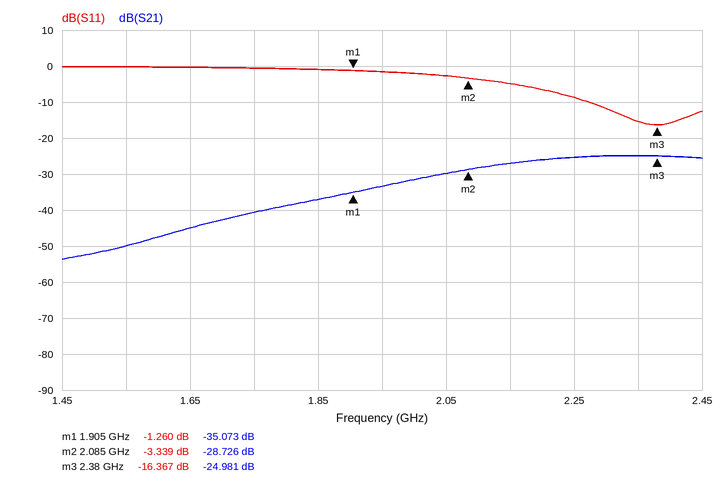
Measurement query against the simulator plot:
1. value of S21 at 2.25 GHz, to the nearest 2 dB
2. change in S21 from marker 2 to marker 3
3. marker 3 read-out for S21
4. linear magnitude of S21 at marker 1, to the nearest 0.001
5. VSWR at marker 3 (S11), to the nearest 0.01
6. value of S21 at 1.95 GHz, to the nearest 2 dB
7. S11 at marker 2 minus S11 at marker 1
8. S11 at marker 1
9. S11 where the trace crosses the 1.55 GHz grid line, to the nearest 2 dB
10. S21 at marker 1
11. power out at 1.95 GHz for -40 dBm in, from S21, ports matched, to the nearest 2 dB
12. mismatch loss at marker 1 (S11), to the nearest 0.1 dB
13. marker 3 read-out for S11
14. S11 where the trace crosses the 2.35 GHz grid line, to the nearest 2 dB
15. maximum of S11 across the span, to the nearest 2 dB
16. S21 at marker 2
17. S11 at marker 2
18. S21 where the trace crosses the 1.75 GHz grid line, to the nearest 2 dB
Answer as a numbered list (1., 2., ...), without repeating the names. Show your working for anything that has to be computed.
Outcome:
1. -26 dB
2. -24.981 − (-28.726) = 3.745 dB
3. -24.981 dB
4. 10^(-35.073/20) ≈ 0.018
5. (1 + 0.1519)/(1 − 0.1519) ≈ 1.36
6. -34 dB
7. -3.339 − (-1.26) = -2.079 dB
8. -1.260 dB
9. 0 dB
10. -35.073 dB
11. -40 dBm + (-34 dB) = -74 dBm
12. −10 log10(1 − 10^(-1.26/10)) ≈ 6.0 dB
13. -16.367 dB
14. -16 dB
15. 0 dB
16. -28.726 dB
17. -3.339 dB
18. -40 dB
